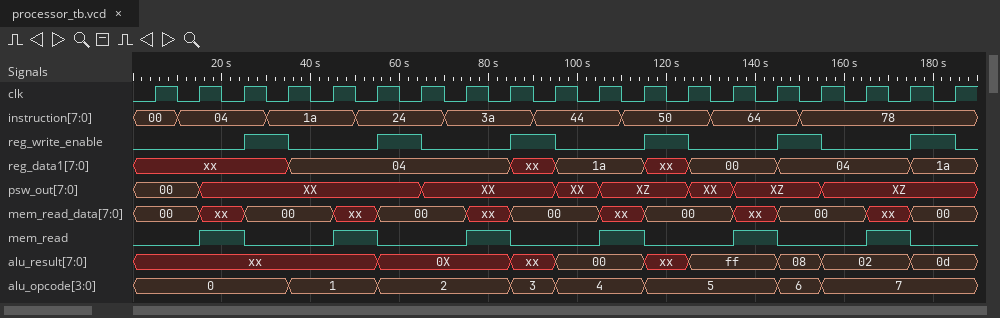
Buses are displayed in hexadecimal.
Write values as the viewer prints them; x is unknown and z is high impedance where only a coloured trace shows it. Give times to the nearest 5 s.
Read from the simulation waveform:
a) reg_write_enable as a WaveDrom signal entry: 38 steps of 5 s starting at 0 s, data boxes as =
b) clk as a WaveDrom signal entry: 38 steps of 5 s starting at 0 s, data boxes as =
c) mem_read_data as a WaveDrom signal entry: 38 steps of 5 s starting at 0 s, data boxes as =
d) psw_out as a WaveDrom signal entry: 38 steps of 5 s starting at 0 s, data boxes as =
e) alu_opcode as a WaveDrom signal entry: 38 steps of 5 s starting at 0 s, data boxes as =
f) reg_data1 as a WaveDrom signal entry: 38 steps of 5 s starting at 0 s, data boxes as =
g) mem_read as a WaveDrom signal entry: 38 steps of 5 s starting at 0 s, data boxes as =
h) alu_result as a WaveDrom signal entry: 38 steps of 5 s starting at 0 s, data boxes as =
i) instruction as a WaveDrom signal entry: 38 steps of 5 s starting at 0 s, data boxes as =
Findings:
{name: 'reg_write_enable', wave: '0....1.0...1.0...1.0...1.0...1.0...1.0'}
{name: 'clk', wave: '01010101010101010101010101010101010101'}
{name: 'mem_read_data', wave: '=..x.=...x.=...x.=...x.=...x.=...x.=..', data: '00 00 00 00 00 00 00'}
{name: 'psw_out', wave: '=..=.........=.....=.=...=.=...=......', data: '00 XX XX XX XZ XX XZ XZ'}
{name: 'alu_opcode', wave: '=......=...=.....=.=...=.....=.=......', data: '0 1 2 3 4 5 6 7'}
{name: 'reg_data1', wave: 'x......=.........x.=...x.=...=.....=..', data: '04 1a 00 04 1a'}
{name: 'mem_read', wave: '0..1.0...1.0...1.0...1.0...1.0...1.0..'}
{name: 'alu_result', wave: 'x..........=.....x.=...x.=...=.=...=..', data: '0X 00 ff 08 02 0d'}
{name: 'instruction', wave: '=.=...=...=...=...=...=...=...=.......', data: '00 04 1a 24 3a 44 50 64 78'}
